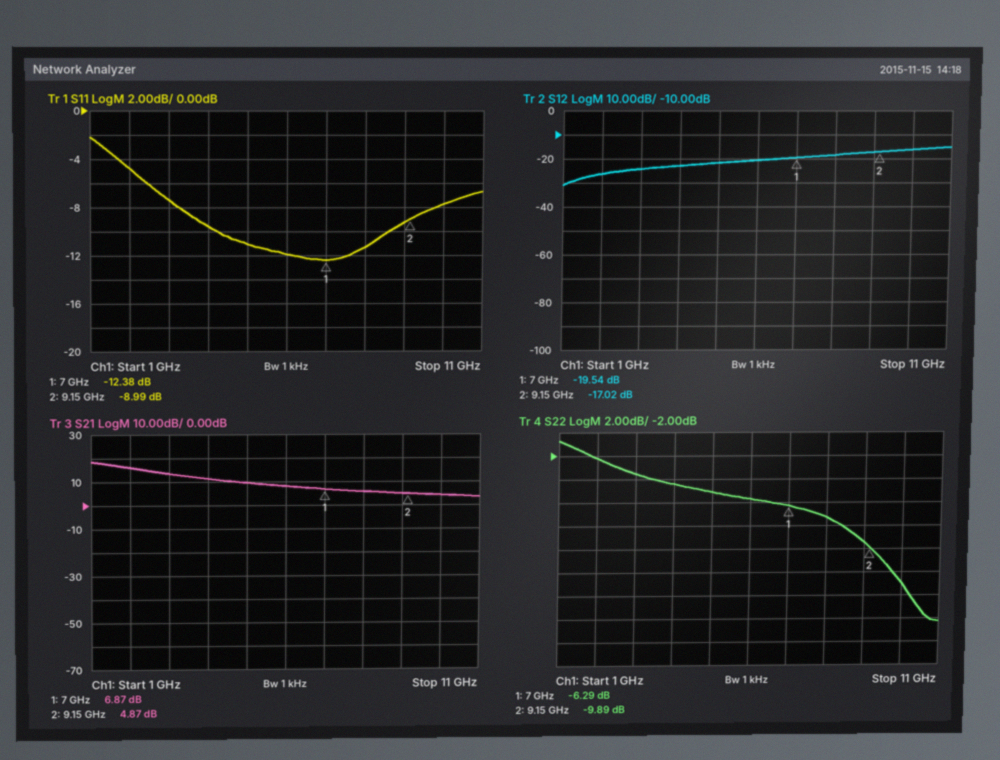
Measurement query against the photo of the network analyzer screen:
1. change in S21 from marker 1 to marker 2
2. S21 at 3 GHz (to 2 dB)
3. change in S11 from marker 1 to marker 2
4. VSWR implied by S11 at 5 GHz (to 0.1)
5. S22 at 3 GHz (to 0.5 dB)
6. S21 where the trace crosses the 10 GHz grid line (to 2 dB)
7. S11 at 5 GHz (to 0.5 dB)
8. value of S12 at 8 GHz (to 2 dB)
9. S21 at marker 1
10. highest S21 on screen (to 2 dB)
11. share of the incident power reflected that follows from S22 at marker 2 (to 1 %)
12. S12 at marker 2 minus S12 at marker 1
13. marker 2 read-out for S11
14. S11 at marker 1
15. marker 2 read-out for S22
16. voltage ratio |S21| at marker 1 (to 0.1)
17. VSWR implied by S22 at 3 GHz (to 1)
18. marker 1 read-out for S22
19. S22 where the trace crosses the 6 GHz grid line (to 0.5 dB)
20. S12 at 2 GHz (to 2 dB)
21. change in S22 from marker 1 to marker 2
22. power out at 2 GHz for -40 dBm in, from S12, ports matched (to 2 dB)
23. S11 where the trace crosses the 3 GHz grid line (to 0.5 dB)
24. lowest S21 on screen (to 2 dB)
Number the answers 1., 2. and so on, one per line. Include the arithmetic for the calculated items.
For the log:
1. 4.87 − (6.87) = -2.00 dB
2. 14 dB
3. -8.99 − (-12.38) = 3.39 dB
4. |Γ| = 10^(-11/20) = 0.2818; VSWR = (1 + 0.2818)/(1 − 0.2818) ≈ 1.8
5. -3.5 dB
6. 4 dB
7. -11.0 dB
8. -18 dB
9. 6.87 dB
10. 18 dB
11. 10^(-9.89/10) ≈ 10 %
12. -17.02 − (-19.54) = 2.52 dB
13. -8.99 dB
14. -12.38 dB
15. -9.89 dB
16. 10^(6.87/20) ≈ 2.2
17. |Γ| = 10^(-3.5/20) = 0.6683; VSWR = (1 + 0.6683)/(1 − 0.6683) ≈ 5
18. -6.29 dB
19. -5.5 dB
20. -26 dB
21. -9.89 − (-6.29) = -3.60 dB
22. -40 dBm + (-26 dB) = -66 dBm
23. -7.5 dB
24. 4 dB
